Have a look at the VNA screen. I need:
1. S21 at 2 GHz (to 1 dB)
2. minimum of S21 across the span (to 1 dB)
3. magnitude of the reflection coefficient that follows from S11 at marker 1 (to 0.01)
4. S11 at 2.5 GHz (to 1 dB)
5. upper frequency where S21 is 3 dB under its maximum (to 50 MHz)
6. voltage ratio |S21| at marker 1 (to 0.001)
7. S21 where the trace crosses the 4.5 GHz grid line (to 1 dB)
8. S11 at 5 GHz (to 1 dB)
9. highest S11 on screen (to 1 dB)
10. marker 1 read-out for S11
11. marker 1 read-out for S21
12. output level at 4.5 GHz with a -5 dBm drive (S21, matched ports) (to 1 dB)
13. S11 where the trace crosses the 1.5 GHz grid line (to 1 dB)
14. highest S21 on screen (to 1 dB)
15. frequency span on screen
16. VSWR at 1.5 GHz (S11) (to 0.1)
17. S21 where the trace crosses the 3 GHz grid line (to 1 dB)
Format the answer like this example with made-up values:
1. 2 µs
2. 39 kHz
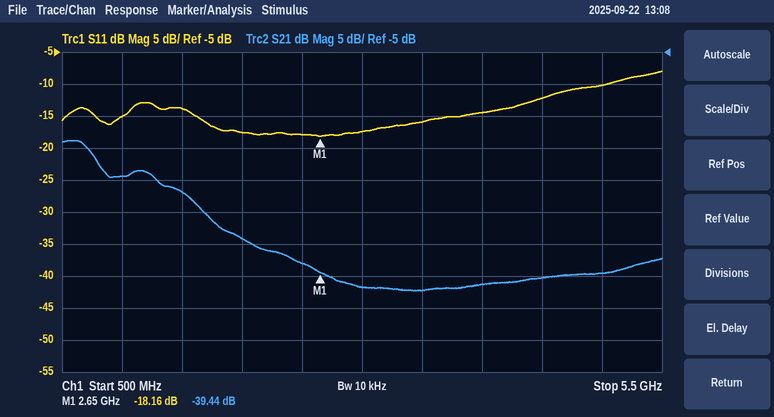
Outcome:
1. -34 dB
2. -42 dB
3. 0.12
4. -18 dB
5. 800 MHz
6. 0.011
7. -40 dB
8. -10 dB
9. -8 dB
10. -18.16 dB
11. -39.44 dB
12. -45 dBm
13. -14 dB
14. -19 dB
15. 5 GHz
16. 1.5
17. -42 dB
